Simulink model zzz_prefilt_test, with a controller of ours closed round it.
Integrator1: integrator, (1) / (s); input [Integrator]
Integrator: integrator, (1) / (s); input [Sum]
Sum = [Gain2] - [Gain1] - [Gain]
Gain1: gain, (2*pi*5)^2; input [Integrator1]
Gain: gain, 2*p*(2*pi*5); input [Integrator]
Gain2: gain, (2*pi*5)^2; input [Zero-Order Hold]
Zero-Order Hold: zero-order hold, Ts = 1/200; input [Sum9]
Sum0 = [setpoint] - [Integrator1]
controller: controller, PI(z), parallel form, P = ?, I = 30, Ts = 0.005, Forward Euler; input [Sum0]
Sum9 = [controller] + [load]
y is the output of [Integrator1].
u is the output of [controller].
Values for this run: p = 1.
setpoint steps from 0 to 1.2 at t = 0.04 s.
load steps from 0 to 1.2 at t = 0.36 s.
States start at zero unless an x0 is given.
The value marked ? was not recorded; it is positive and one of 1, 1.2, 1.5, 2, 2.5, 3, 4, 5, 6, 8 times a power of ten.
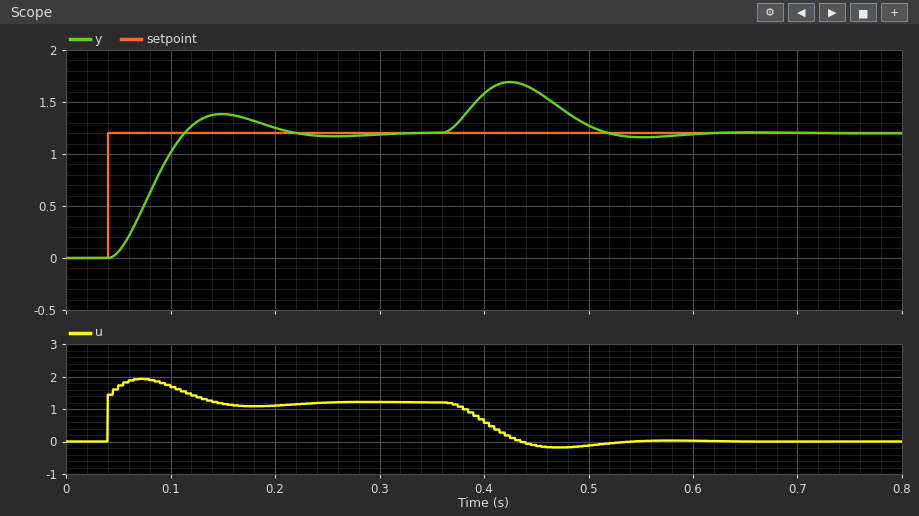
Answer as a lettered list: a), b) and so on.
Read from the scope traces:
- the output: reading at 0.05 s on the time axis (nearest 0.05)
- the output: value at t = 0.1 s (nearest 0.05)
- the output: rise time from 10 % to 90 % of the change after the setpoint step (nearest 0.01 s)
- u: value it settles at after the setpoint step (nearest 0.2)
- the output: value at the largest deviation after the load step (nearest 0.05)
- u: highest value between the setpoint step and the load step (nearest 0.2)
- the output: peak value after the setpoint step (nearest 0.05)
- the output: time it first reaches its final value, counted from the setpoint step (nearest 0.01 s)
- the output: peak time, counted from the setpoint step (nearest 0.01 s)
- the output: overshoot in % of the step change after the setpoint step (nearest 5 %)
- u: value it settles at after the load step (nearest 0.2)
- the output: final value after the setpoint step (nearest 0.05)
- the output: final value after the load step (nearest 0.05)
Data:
a) 0.05
b) 1.00
c) 0.05 s
d) 1.2
e) 1.70
f) 2.0
g) 1.40
h) 0.07 s
i) 0.11 s
j) 15 %
k) 0.0
l) 1.20
m) 1.20
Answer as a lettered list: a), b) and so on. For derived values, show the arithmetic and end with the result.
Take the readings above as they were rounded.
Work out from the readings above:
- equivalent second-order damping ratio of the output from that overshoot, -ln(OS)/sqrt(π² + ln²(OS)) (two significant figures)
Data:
a) ln(0.15) = -1.897; 1.897 / sqrt(9.870 + 3.599) = 0.52
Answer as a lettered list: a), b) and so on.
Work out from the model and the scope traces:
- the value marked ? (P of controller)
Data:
a) 1.2
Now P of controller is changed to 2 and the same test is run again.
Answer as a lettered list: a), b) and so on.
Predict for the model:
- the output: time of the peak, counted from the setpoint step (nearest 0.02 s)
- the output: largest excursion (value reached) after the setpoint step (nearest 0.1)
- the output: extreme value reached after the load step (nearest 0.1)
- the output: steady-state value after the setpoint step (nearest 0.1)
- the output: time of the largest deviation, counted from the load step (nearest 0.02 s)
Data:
a) 0.08 s
b) 1.3
c) 1.6
d) 1.2
e) 0.06 s
